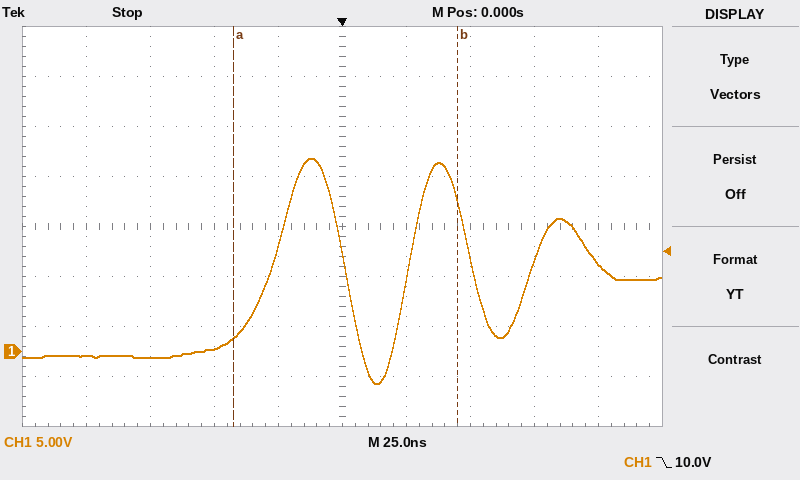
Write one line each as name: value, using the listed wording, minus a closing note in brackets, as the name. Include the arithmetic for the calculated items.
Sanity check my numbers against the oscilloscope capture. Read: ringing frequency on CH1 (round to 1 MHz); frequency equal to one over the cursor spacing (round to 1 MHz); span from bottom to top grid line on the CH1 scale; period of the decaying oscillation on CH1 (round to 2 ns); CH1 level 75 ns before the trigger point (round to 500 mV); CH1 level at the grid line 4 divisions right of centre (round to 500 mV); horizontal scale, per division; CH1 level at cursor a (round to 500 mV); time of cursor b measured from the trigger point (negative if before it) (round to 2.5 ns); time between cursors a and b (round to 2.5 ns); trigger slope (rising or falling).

ringing frequency on CH1: 1 / 48 ns ≈ 21 MHz
frequency equal to one over the cursor spacing: 1 / 87.5 ns ≈ 11 MHz
span from bottom to top grid line on the CH1 scale: 40 V
period of the decaying oscillation on CH1: 48 ns
CH1 level 75 ns before the trigger point: -500 mV
CH1 level at the grid line 4 divisions right of centre: 9.0 V
horizontal scale, per division: 25 ns
CH1 level at cursor a: 1.5 V
time of cursor b measured from the trigger point (negative if before it): +45.0 ns
time between cursors a and b: 87.5 ns
trigger slope: falling
